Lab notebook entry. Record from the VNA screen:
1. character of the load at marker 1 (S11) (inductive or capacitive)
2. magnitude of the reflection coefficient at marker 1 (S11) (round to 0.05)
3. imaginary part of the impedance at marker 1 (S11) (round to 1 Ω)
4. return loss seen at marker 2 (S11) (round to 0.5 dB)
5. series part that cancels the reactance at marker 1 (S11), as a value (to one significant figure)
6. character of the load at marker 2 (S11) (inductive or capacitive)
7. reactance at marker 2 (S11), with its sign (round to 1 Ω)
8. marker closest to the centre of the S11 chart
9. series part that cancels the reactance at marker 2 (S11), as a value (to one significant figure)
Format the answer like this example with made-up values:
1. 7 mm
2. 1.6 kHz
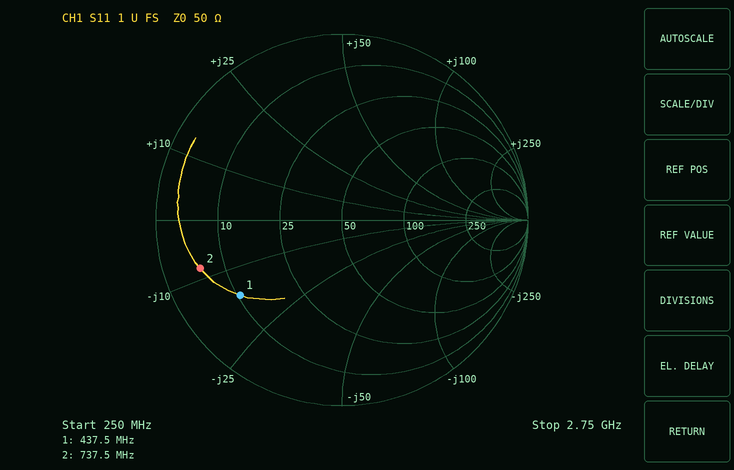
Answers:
1. capacitive
2. 0.70
3. -16 Ω
4. 2.0 dB
5. 6 nH
6. capacitive
7. -8 Ω
8. marker 1
9. 2 nH
